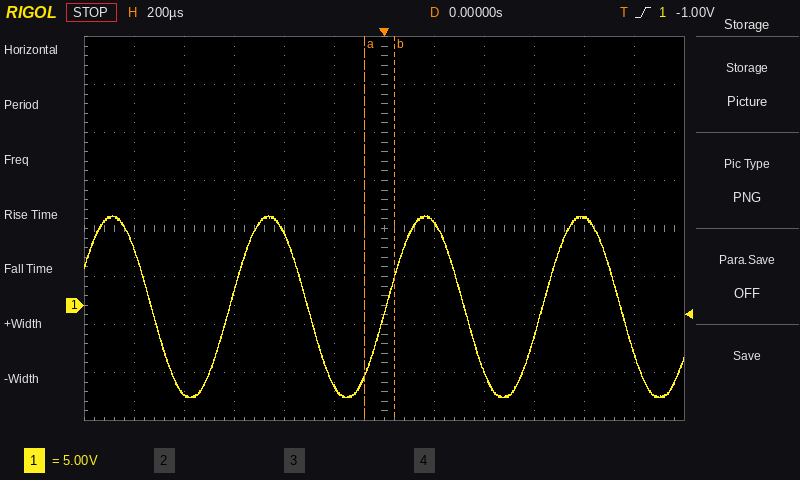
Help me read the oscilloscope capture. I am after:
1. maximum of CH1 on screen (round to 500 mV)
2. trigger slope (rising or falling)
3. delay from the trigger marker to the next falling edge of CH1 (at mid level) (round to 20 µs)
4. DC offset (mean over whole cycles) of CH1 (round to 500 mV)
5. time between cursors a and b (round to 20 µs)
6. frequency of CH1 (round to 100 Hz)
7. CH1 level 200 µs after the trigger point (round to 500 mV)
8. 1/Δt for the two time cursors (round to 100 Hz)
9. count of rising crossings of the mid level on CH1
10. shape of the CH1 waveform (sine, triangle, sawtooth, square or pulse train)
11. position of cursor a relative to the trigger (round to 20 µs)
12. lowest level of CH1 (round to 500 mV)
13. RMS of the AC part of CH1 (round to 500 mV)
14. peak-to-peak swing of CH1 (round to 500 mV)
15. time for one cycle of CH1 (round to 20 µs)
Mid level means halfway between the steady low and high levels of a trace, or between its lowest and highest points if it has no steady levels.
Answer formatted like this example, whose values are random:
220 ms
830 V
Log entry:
9.5 V
rising
320 µs
0.0 V
120 µs
1.6 kHz
8.5 V
8.3 kHz
3
sine
-80 µs
-9.5 V
6.5 V
19.0 V
620 µs
